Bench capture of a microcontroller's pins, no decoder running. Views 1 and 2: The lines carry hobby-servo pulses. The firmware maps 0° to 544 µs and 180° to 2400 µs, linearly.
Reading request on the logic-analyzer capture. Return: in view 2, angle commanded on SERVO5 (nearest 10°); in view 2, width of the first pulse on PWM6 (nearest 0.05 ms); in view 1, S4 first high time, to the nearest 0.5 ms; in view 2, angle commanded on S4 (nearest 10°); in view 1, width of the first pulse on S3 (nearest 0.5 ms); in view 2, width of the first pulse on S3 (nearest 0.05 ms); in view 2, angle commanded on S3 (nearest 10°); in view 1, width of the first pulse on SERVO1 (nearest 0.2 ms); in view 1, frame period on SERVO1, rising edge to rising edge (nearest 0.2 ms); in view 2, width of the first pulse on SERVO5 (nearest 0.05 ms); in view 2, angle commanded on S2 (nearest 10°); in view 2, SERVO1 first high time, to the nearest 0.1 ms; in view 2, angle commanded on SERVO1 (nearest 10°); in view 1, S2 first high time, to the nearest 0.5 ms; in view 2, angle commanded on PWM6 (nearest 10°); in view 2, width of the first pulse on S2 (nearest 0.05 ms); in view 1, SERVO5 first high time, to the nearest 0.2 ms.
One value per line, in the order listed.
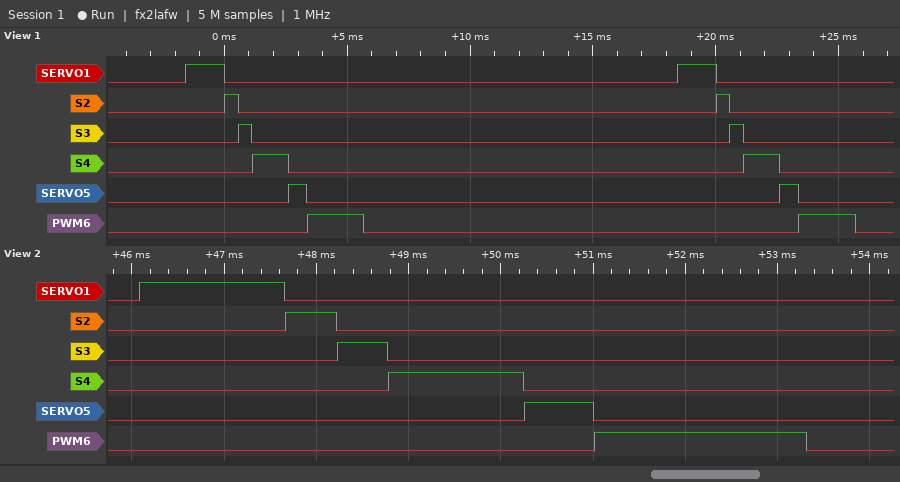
20°
2.30 ms
1.5 ms
90°
0.5 ms
0.55 ms
0°
1.6 ms
20.0 ms
0.75 ms
0°
1.6 ms
100°
0.5 ms
170°
0.55 ms
0.8 ms
